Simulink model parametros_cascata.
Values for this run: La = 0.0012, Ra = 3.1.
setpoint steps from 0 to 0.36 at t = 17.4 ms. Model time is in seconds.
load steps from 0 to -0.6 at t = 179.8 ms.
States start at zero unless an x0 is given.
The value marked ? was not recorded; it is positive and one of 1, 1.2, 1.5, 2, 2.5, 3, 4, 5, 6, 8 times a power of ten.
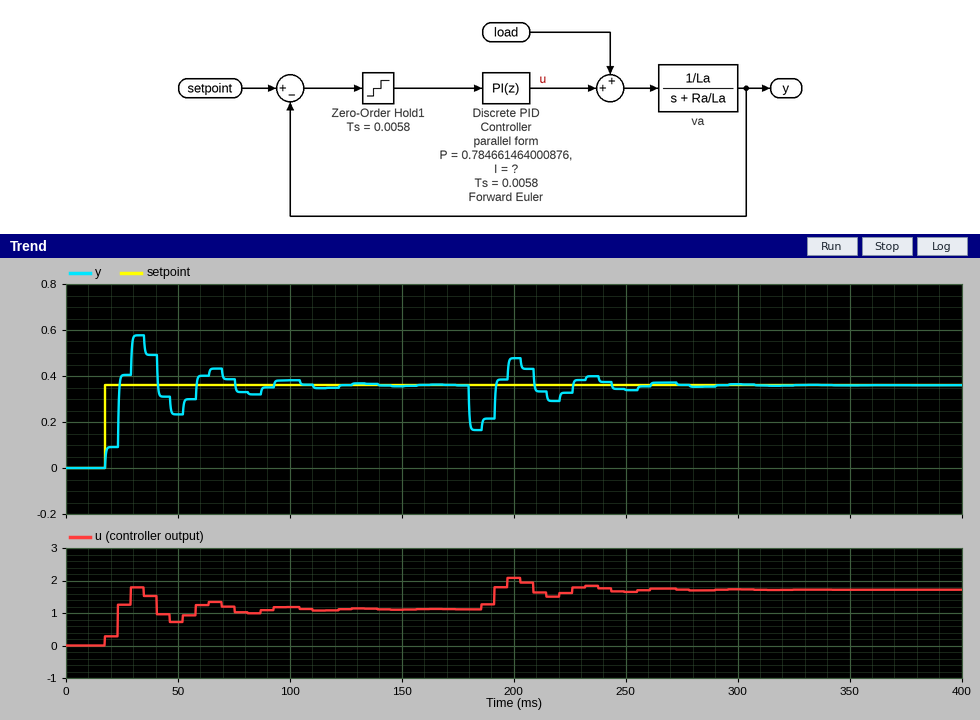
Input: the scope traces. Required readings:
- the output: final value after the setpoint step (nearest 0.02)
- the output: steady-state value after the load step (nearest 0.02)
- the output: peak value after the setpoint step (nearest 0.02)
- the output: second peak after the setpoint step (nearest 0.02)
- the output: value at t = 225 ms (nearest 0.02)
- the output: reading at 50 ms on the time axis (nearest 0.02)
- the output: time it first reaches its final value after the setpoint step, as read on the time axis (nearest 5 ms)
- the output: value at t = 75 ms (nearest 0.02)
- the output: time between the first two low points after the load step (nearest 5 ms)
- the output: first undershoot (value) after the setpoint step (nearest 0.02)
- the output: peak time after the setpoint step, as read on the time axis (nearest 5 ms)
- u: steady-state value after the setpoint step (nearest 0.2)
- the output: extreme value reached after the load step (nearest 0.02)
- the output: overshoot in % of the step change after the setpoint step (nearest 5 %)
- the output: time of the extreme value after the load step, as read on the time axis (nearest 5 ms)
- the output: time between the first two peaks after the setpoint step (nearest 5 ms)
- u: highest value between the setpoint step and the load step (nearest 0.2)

0.36
0.36
0.58
0.44
0.32
0.24
25 ms
0.38
35 ms
0.24
35 ms
1.2
0.16
60 %
185 ms
35 ms
1.8
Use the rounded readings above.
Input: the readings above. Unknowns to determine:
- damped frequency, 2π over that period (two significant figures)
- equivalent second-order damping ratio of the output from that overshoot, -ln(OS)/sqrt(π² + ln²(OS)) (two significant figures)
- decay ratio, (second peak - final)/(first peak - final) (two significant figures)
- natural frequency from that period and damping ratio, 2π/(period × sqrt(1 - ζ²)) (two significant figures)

0.18 rad/ms
0.16
0.36
0.18 rad/ms
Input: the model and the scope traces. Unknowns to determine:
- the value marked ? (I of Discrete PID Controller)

500
